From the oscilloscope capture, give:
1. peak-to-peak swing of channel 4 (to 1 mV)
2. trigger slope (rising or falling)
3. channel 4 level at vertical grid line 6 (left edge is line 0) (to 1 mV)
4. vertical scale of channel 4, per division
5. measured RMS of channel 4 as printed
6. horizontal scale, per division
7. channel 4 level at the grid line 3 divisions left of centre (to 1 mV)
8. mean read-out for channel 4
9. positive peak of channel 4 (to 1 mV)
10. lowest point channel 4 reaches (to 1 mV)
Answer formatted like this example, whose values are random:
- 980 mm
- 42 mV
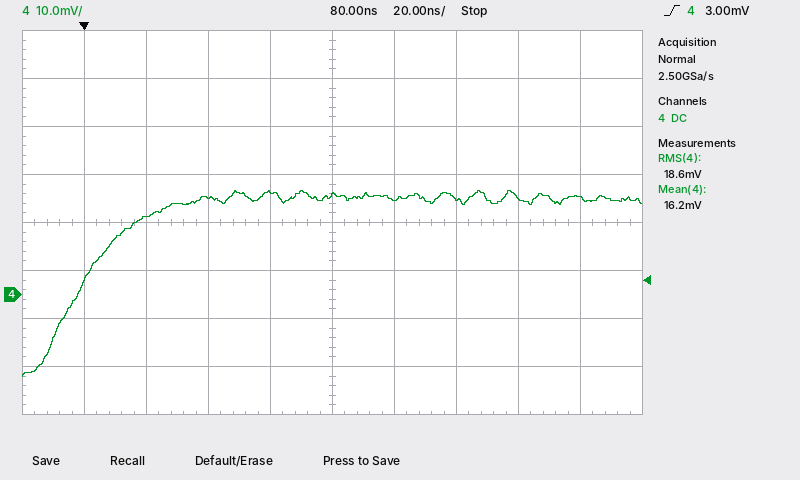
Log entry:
- 39 mV
- rising
- 20 mV
- 10 mV
- 18.6 mV
- 20 ns
- 16 mV
- 16.2 mV
- 22 mV
- -17 mV
